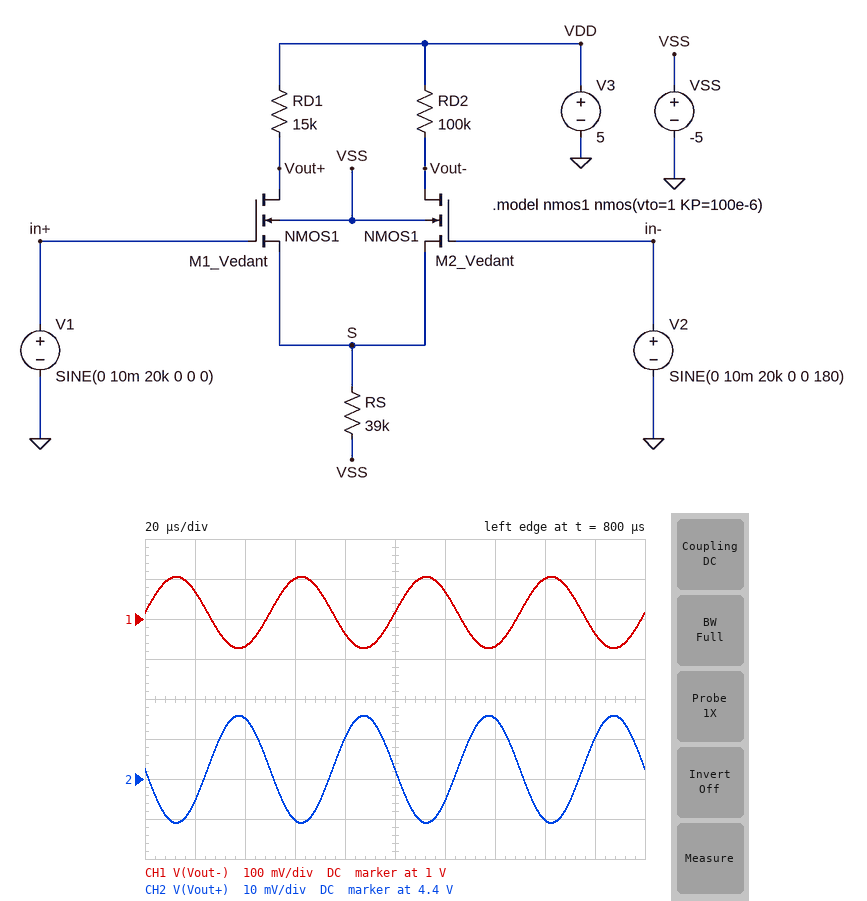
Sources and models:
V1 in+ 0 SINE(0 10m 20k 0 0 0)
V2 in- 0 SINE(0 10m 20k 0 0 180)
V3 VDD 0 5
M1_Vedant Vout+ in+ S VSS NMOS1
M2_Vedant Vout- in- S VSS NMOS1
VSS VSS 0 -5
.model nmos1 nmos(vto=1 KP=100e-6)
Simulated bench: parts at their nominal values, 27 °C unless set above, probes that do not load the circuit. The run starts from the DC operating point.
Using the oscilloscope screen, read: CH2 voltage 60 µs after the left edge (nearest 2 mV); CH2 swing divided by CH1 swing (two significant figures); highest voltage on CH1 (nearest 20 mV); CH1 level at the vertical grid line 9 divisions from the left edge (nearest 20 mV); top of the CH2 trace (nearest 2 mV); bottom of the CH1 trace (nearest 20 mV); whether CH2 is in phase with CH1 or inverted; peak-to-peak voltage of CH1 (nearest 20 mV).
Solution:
4.390 V
0.15
1.10 V
960 mV
4.416 V
920 mV
inverted
180 mV
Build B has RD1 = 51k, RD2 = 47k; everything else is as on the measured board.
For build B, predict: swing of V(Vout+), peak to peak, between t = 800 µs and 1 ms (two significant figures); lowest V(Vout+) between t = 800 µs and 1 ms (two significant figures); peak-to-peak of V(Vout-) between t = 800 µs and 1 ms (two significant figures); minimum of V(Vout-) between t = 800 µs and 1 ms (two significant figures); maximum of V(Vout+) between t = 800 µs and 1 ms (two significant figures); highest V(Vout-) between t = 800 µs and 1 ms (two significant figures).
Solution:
91 mV
2.9 V
84 mV
3.1 V
3.0 V
3.2 V
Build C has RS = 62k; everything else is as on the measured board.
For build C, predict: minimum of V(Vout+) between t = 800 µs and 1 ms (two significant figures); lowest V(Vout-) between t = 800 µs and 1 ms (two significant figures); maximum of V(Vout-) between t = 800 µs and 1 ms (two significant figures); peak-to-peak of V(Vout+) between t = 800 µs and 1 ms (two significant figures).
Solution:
4.6 V
2.3 V
2.4 V
22 mV
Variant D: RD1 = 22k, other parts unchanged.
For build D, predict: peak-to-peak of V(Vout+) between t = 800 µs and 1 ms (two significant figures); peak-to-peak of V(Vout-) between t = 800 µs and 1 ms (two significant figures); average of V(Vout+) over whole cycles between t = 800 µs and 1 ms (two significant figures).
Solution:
39 mV
180 mV
4.1 V
